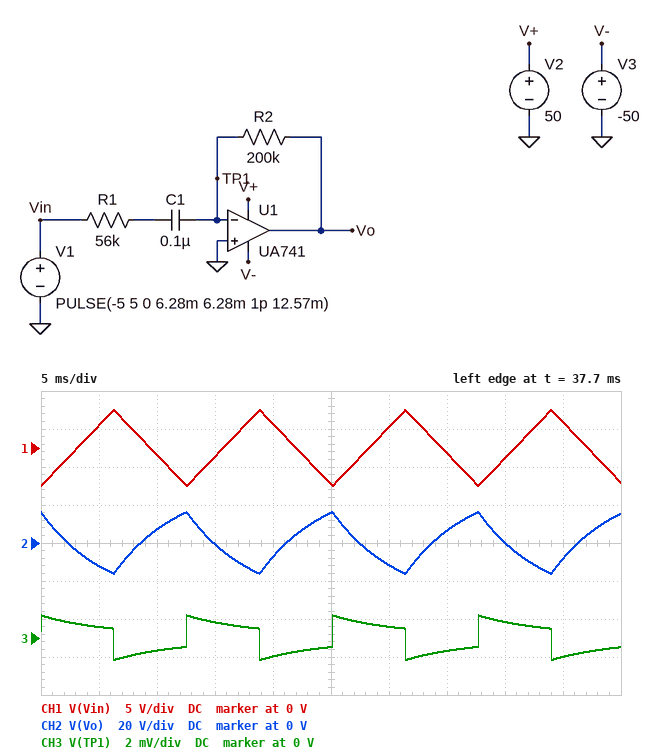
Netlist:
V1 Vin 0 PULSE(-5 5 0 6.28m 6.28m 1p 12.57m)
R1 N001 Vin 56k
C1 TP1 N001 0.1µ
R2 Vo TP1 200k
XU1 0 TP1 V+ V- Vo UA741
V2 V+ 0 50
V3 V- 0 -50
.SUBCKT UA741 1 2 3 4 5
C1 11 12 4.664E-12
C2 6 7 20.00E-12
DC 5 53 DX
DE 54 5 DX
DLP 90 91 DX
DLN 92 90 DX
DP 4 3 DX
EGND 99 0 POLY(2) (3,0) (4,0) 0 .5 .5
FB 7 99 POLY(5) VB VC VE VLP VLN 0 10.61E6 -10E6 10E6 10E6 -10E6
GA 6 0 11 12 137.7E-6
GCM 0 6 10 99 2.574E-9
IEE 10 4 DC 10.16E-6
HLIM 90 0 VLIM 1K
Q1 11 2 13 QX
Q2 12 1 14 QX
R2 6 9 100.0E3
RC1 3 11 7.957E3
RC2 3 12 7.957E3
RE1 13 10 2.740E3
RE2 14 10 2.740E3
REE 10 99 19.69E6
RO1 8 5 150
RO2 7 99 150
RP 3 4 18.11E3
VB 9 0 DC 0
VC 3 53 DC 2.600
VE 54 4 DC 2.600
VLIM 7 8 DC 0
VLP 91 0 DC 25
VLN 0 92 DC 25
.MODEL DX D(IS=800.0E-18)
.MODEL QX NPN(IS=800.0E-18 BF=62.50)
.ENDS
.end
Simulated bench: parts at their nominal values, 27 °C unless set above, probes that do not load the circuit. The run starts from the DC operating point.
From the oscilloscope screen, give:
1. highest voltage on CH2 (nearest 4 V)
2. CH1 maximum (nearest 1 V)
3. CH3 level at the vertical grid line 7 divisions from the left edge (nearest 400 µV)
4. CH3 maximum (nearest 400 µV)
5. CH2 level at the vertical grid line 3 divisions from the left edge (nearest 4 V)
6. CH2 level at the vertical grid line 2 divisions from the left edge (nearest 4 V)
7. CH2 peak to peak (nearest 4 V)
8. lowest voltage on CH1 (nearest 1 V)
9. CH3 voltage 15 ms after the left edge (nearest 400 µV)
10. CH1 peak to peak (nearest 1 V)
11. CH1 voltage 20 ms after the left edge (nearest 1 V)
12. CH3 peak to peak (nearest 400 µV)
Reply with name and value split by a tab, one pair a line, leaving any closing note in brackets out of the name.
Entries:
highest voltage on CH2	16 V
CH1 maximum	5 V
CH3 level at the vertical grid line 7 divisions from the left edge	-800 µV
CH3 maximum	1.2 mV
CH2 level at the vertical grid line 3 divisions from the left edge	0 V
CH2 level at the vertical grid line 2 divisions from the left edge	8 V
CH2 peak to peak	32 V
lowest voltage on CH1	-5 V
CH3 voltage 15 ms after the left edge	800 µV
CH1 peak to peak	10 V
CH1 voltage 20 ms after the left edge	3 V
CH3 peak to peak	2.4 mV
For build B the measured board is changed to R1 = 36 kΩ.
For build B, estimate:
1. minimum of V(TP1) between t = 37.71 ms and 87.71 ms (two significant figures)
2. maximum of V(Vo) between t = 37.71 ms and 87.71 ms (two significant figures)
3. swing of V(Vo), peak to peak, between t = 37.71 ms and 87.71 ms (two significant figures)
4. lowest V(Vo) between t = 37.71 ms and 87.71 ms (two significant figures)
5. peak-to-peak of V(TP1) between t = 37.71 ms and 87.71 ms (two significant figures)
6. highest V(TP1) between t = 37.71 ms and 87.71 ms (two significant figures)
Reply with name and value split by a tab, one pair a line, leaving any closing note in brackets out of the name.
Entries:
minimum of V(TP1) between t = 37.71 ms and 87.71 ms	-2.1 mV
maximum of V(Vo) between t = 37.71 ms and 87.71 ms	22 V
swing of V(Vo), peak to peak, between t = 37.71 ms and 87.71 ms	45 V
lowest V(Vo) between t = 37.71 ms and 87.71 ms	-22 V
peak-to-peak of V(TP1) between t = 37.71 ms and 87.71 ms	4.2 mV
highest V(TP1) between t = 37.71 ms and 87.71 ms	2.1 mV
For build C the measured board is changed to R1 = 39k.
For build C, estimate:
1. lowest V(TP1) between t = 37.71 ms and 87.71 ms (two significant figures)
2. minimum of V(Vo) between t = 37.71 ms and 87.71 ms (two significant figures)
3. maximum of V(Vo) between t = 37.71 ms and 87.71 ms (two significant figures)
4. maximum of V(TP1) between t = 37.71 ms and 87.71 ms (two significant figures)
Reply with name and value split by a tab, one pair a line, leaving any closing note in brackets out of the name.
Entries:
lowest V(TP1) between t = 37.71 ms and 87.71 ms	-1.9 mV
minimum of V(Vo) between t = 37.71 ms and 87.71 ms	-21 V
maximum of V(Vo) between t = 37.71 ms and 87.71 ms	21 V
maximum of V(TP1) between t = 37.71 ms and 87.71 ms	1.9 mV
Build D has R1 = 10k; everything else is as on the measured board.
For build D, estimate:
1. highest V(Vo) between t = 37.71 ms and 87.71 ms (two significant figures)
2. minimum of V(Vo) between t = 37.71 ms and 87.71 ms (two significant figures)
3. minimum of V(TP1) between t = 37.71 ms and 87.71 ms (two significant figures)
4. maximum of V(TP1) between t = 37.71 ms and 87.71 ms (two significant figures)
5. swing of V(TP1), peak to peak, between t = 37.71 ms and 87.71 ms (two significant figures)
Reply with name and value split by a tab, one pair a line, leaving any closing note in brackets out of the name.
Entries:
highest V(Vo) between t = 37.71 ms and 87.71 ms	32 V
minimum of V(Vo) between t = 37.71 ms and 87.71 ms	-32 V
minimum of V(TP1) between t = 37.71 ms and 87.71 ms	-9.0 mV
maximum of V(TP1) between t = 37.71 ms and 87.71 ms	9.0 mV
swing of V(TP1), peak to peak, between t = 37.71 ms and 87.71 ms	18 mV
